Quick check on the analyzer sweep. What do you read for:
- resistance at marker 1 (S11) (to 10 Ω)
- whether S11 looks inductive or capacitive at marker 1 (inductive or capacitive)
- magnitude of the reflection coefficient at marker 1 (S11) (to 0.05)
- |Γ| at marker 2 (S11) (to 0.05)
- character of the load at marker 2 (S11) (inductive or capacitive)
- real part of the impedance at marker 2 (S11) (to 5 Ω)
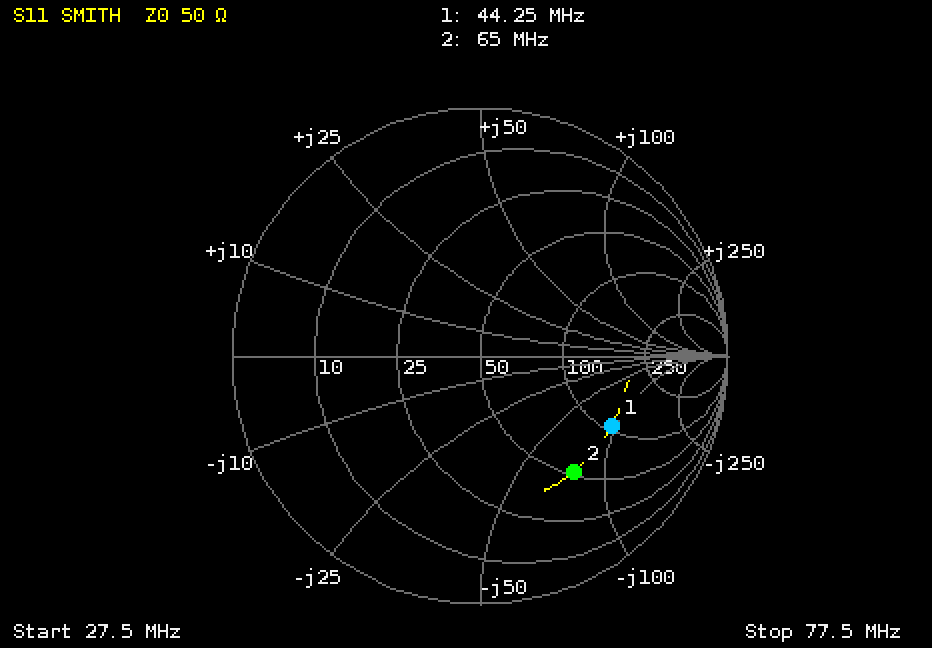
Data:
110 Ω
capacitive
0.60
0.60
capacitive
55 Ω
